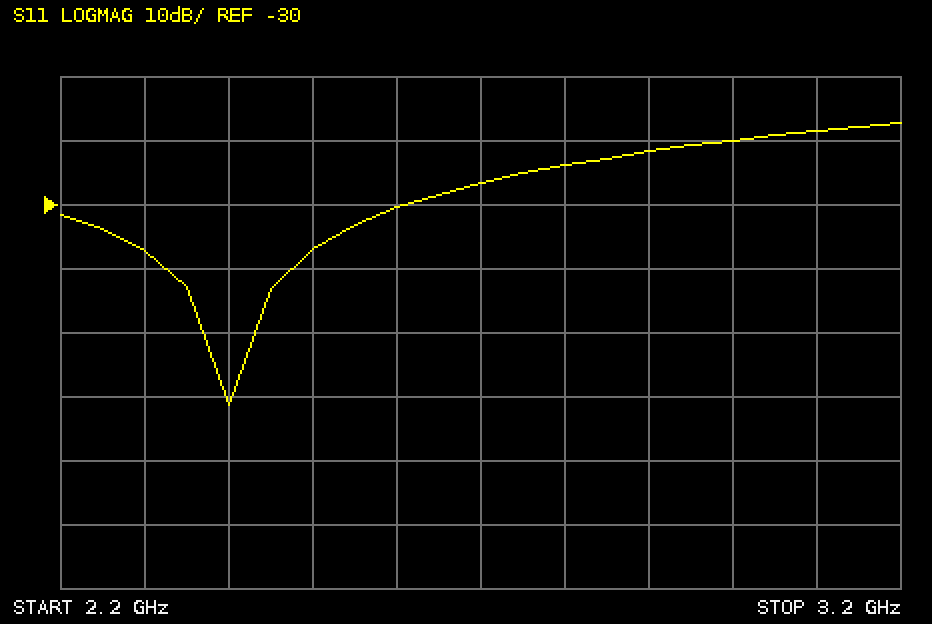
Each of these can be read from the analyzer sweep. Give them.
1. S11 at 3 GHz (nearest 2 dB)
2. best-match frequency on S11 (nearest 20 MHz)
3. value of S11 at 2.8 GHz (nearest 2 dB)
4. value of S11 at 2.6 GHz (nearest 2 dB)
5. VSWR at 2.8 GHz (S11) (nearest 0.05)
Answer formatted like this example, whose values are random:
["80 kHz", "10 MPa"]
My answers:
["-20 dB", "2.40 GHz", "-24 dB", "-30 dB", "1.15"]
